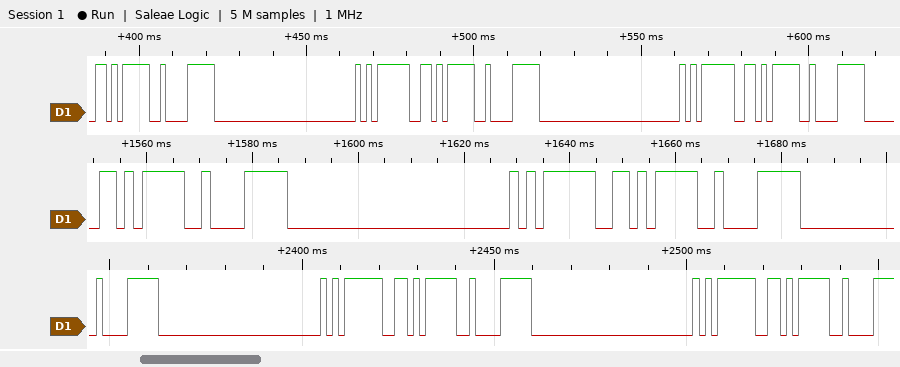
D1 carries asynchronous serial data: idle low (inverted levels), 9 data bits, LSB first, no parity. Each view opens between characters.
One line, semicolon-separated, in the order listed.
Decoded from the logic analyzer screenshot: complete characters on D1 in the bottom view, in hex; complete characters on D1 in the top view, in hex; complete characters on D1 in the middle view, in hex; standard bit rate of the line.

0F, 05, 0A, 0F, 05, 0A; 0A, 0F, 05, 0A, 0F, 05, 0A, 0F; 0A, 0F, 05, 0A, 0F; 600 baud
